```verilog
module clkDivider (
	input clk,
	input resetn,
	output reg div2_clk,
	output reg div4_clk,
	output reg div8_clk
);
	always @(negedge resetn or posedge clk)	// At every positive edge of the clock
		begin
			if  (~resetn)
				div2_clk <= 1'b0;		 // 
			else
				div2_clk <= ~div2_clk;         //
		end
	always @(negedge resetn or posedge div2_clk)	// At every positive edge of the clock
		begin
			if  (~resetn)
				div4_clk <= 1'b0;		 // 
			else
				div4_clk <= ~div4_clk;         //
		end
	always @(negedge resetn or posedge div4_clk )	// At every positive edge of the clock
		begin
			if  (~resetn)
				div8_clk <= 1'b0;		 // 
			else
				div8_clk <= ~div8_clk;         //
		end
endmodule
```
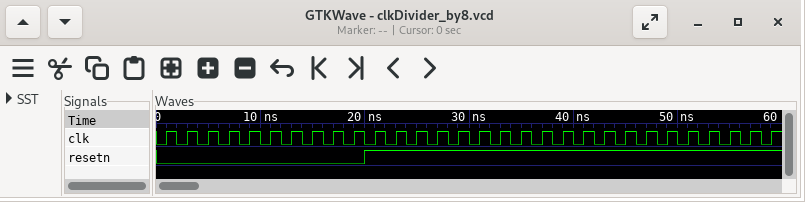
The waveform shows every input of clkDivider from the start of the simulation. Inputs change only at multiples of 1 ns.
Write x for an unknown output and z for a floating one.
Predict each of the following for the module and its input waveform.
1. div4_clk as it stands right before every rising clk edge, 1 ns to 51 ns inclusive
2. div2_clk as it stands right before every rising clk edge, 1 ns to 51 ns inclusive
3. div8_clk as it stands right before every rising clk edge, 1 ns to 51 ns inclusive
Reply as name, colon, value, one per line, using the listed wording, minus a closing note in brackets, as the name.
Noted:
div4_clk as it stands right before every rising clk edge, 1 ns to 51 ns inclusive: 0 0 0 0 0 0 0 0 0 0 0 1 1 0 0 1 1 0 0 1 1 0 0 1 1 0
div2_clk as it stands right before every rising clk edge, 1 ns to 51 ns inclusive: 0 0 0 0 0 0 0 0 0 0 0 1 0 1 0 1 0 1 0 1 0 1 0 1 0 1
div8_clk as it stands right before every rising clk edge, 1 ns to 51 ns inclusive: 0 0 0 0 0 0 0 0 0 0 0 1 1 1 1 0 0 0 0 1 1 1 1 0 0 0
